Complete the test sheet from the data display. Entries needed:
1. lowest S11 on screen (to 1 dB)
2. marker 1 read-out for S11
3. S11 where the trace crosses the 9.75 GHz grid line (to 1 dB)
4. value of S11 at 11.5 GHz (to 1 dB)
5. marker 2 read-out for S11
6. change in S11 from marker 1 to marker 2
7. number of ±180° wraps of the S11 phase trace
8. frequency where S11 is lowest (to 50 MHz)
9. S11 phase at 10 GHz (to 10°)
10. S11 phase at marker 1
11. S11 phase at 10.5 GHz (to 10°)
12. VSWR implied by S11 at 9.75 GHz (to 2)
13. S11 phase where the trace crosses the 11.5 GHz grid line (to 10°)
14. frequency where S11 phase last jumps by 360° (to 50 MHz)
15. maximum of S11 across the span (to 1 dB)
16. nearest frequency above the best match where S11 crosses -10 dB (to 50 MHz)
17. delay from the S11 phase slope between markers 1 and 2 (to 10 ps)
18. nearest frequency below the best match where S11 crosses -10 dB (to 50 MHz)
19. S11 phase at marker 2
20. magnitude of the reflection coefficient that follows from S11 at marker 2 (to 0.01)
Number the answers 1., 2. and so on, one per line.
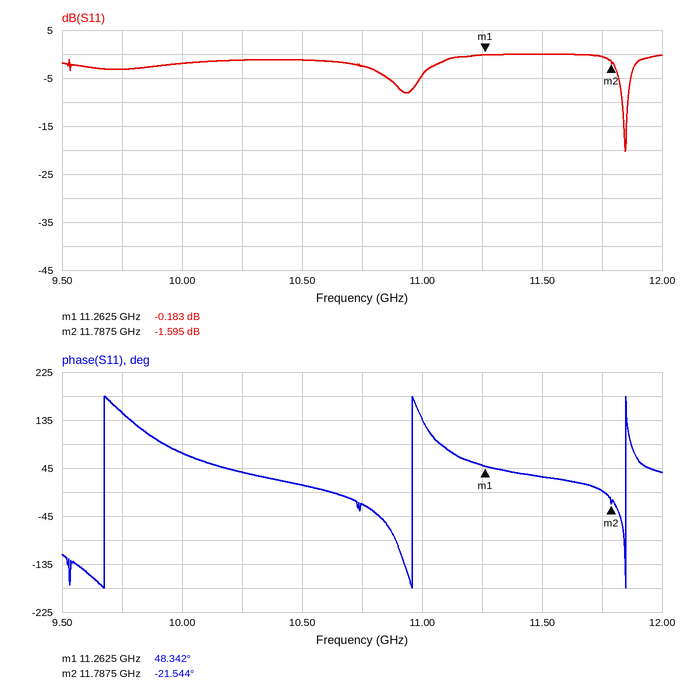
1. -20 dB
2. -0.183 dB
3. -3 dB
4. 0 dB
5. -1.595 dB
6. -1.412 dB
7. 3
8. 11.85 GHz
9. 70°
10. 48.342°
11. 10°
12. 6
13. 30°
14. 11.85 GHz
15. 0 dB
16. 11.85 GHz
17. 370 ps
18. 11.85 GHz
19. -21.544°
20. 0.83
